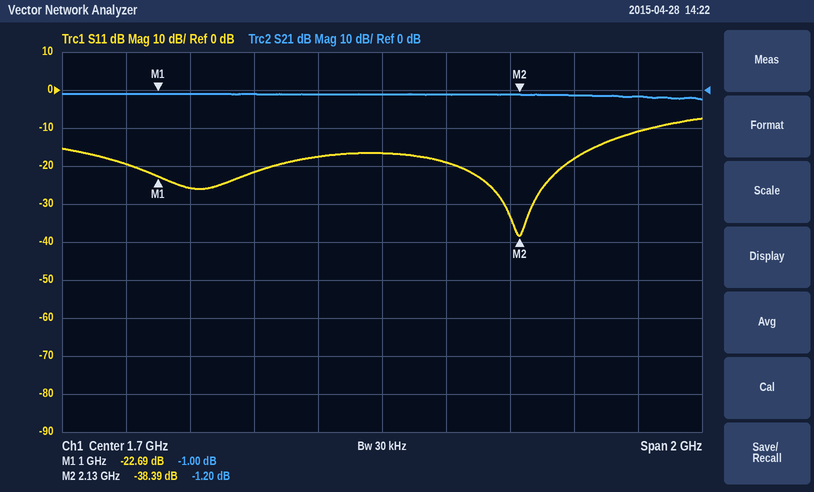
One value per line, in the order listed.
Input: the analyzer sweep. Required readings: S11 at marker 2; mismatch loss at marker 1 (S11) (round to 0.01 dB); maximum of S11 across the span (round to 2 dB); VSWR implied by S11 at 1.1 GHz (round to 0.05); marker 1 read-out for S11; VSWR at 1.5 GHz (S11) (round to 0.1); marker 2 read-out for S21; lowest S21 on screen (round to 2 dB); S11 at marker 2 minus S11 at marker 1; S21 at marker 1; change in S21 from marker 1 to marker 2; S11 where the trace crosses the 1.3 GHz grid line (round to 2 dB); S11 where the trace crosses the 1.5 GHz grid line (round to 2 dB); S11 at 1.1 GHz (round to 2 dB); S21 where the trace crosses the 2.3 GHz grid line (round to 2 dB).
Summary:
-38.39 dB
0.02 dB
-8 dB
1.10
-22.69 dB
1.3
-1.20 dB
-2 dB
-15.70 dB
-1.00 dB
-0.20 dB
-22 dB
-18 dB
-26 dB
-2 dB
